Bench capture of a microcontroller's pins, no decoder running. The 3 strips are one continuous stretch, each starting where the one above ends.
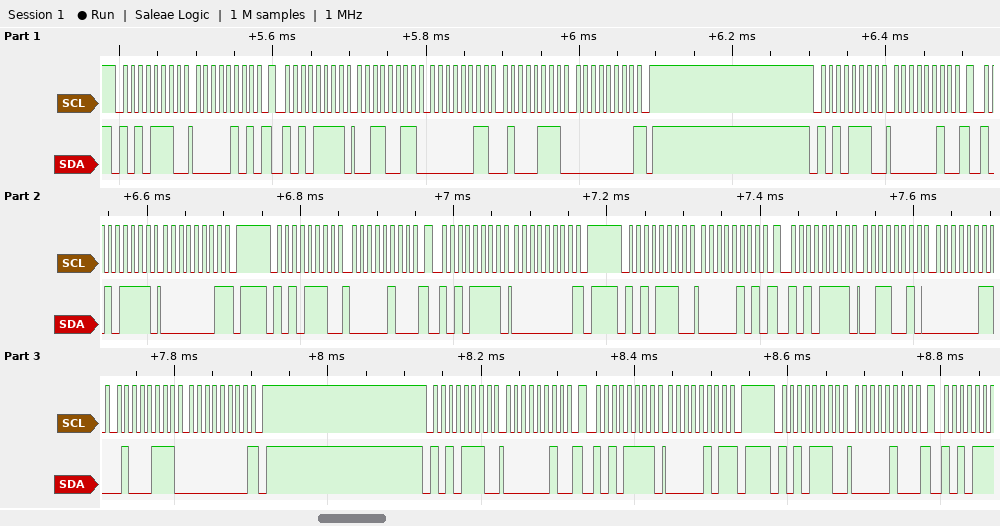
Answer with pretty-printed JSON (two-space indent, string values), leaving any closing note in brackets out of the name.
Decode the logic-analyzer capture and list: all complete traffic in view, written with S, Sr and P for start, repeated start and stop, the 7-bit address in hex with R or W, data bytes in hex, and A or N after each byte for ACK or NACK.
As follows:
{
  "all complete traffic in view, written with S, Sr and P for start, repeated start and stop, the 7-bit address in hex with R or W, data bytes in hex, and A or N after each byte for ACK or NACK": "S 57W A 05 A Sr 57R A 33 A 03 A 47 A 00 N P S 57W A 02 A Sr 57R A 01 N P S 57W A 04 A Sr 57R A 00 N P S 57W A 05 A Sr 57R A 32 A 03 A 47 A 00 N P S 57W A 02 A Sr 57R A 05 N P S 57W A 04 A"
}
